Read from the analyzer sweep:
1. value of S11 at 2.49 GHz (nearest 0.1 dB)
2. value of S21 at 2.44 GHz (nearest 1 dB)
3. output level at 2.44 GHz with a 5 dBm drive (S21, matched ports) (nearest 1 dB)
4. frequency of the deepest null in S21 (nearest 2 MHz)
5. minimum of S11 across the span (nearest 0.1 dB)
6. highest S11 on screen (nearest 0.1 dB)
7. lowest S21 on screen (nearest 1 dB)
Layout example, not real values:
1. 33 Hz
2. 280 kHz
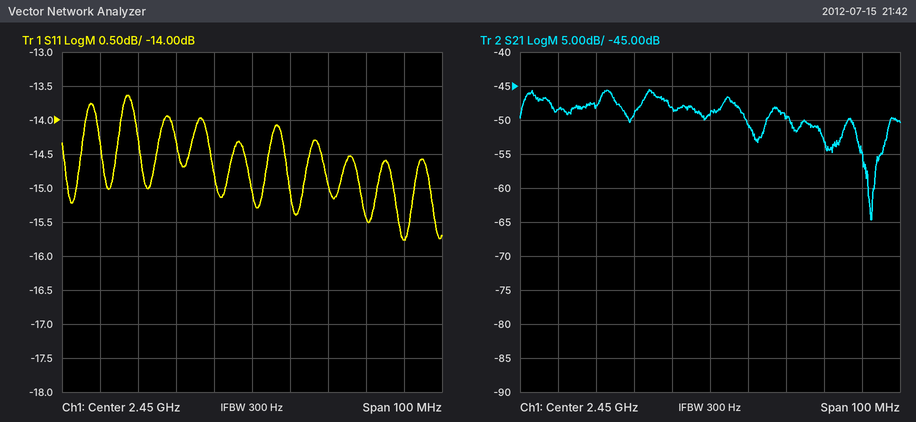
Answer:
1. -15.8 dB
2. -48 dB
3. -43 dBm
4. 2.492 GHz
5. -15.8 dB
6. -13.6 dB
7. -65 dB
